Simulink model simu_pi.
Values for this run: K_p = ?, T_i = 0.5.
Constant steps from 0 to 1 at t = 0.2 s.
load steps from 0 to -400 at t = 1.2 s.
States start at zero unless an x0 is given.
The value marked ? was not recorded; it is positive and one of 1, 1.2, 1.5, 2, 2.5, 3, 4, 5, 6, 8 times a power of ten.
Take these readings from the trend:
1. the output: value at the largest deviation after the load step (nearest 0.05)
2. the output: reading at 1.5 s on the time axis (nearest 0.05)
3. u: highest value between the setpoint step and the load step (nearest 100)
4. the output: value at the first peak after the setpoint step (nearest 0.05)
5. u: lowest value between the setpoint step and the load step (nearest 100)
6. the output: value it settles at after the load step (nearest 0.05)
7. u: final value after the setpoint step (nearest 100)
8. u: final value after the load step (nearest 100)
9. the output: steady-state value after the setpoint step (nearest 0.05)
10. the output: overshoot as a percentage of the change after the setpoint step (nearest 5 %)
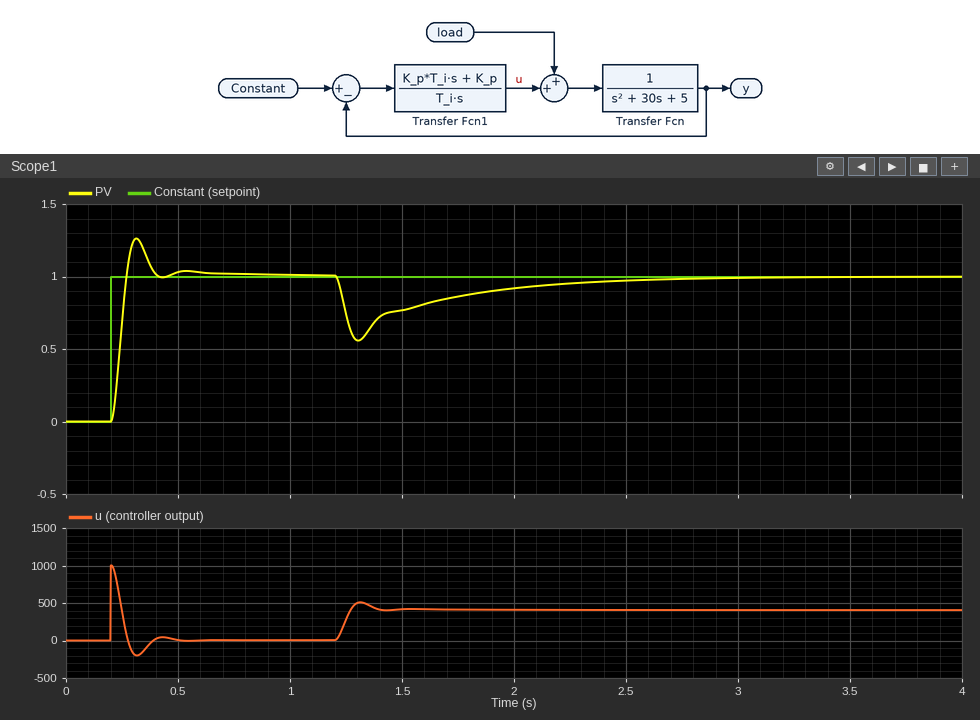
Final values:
0.55
0.75
1000
1.25
-200
1.00
0
400
1.00
25 %
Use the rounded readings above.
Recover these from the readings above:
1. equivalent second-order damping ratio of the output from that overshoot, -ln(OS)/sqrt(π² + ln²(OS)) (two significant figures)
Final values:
0.40
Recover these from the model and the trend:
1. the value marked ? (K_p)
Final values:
1000
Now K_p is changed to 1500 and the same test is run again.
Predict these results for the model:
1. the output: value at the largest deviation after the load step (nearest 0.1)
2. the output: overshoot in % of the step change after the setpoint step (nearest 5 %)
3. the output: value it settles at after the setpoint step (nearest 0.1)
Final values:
0.7
35 %
1.0
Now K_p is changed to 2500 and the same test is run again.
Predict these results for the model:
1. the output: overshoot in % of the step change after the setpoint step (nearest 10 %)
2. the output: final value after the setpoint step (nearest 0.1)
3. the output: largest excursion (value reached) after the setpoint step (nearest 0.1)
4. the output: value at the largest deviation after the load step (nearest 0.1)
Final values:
40 %
1.0
1.4
0.8
